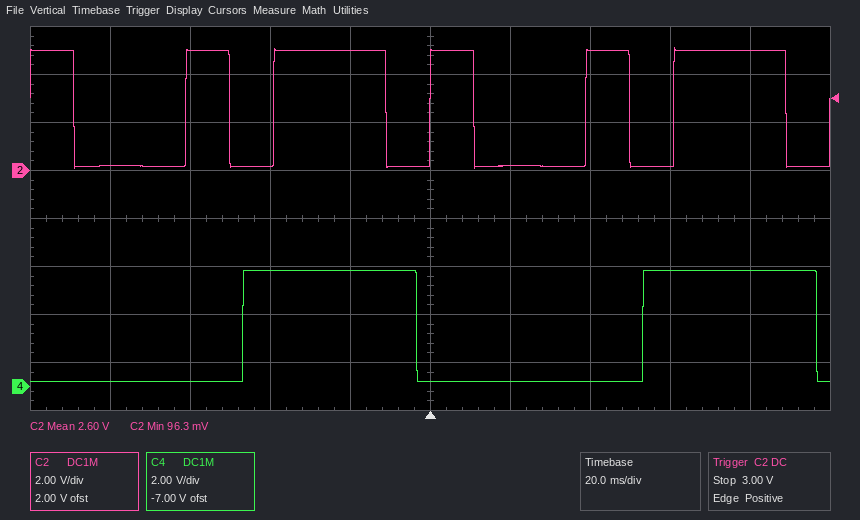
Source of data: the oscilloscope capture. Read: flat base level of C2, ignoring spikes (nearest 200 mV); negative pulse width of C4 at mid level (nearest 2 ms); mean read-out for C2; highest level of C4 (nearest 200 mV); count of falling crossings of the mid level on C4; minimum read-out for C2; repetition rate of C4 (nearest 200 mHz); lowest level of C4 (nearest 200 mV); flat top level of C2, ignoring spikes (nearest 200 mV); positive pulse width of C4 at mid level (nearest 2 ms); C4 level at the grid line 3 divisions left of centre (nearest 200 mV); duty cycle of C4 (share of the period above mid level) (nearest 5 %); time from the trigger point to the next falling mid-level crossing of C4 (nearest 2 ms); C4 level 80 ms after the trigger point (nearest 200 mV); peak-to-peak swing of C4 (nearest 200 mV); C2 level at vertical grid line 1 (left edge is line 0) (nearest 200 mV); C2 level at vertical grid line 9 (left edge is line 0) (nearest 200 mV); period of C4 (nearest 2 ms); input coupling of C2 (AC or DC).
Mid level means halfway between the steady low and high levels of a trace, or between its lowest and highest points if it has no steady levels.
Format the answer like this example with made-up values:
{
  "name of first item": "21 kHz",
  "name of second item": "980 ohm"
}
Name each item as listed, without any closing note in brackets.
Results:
{
  "flat base level of C2, ignoring spikes": "200 mV",
  "negative pulse width of C4 at mid level": "56 ms",
  "mean read-out for C2": "2.60 V",
  "highest level of C4": "4.8 V",
  "count of falling crossings of the mid level on C4": "2",
  "minimum read-out for C2": "96.3 mV",
  "repetition rate of C4": "10.0 Hz",
  "lowest level of C4": "200 mV",
  "flat top level of C2, ignoring spikes": "5.0 V",
  "positive pulse width of C4 at mid level": "44 ms",
  "C4 level at the grid line 3 divisions left of centre": "200 mV",
  "duty cycle of C4 (share of the period above mid level)": "45 %",
  "time from the trigger point to the next falling mid-level crossing of C4": "96 ms",
  "C4 level 80 ms after the trigger point": "4.8 V",
  "peak-to-peak swing of C4": "4.6 V",
  "C2 level at vertical grid line 1 (left edge is line 0)": "200 mV",
  "C2 level at vertical grid line 9 (left edge is line 0)": "5.0 V",
  "period of C4": "100 ms",
  "input coupling of C2": "DC"
}
